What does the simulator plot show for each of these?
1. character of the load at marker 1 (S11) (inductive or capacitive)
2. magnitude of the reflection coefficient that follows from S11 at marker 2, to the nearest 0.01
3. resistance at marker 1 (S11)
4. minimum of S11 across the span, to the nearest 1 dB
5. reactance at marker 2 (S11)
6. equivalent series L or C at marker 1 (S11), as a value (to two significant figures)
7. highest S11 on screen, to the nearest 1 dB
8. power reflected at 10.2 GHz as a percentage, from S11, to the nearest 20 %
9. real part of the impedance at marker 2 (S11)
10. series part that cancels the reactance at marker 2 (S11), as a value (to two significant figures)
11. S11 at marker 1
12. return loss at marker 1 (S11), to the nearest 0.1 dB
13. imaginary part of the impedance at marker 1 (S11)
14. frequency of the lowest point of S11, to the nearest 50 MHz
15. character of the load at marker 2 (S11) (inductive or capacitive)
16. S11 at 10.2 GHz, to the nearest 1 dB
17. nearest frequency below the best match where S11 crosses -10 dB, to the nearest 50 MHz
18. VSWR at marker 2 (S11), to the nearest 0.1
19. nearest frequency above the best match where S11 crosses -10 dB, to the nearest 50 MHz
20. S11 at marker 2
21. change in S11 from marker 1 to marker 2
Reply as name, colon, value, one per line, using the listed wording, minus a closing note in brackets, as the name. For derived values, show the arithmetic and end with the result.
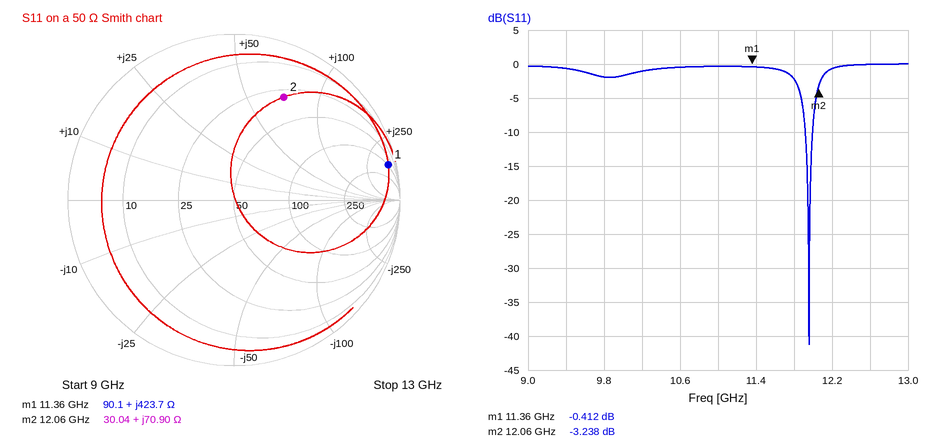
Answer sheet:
character of the load at marker 1 (S11): inductive
magnitude of the reflection coefficient that follows from S11 at marker 2, to the nearest 0.01: 10^(-3.238/20) ≈ 0.69
resistance at marker 1: 90.1 Ω
minimum of S11 across the span, to the nearest 1 dB: -41 dB
reactance at marker 2: +70.90 Ω
equivalent series L or C at marker 1 (S11), as a value: L = 423.7 Ω/(2π × 11.36 GHz) ≈ 5.9 nH
highest S11 on screen, to the nearest 1 dB: 0 dB
power reflected at 10.2 GHz as a percentage, from S11, to the nearest 20 %: 10^(-1/10) ≈ 79.4 %, so 80 % to the nearest 20 %
real part of the impedance at marker 2: 30.04 Ω
series part that cancels the reactance at marker 2 (S11), as a value: C = 1/(2π × 12.06 GHz × 70.9 Ω) ≈ 186 fF, so 190 fF to two significant figures
S11 at marker 1: -0.412 dB
return loss at marker 1 (S11), to the nearest 0.1 dB: 0.4 dB
imaginary part of the impedance at marker 1: +423.7 Ω
frequency of the lowest point of S11, to the nearest 50 MHz: 11.95 GHz
character of the load at marker 2 (S11): inductive
S11 at 10.2 GHz, to the nearest 1 dB: -1 dB
nearest frequency below the best match where S11 crosses -10 dB, to the nearest 50 MHz: 11.90 GHz
VSWR at marker 2 (S11), to the nearest 0.1: 5.4
nearest frequency above the best match where S11 crosses -10 dB, to the nearest 50 MHz: 12.00 GHz
S11 at marker 2: -3.238 dB
change in S11 from marker 1 to marker 2: -3.238 − (-0.412) = -2.826 dB
